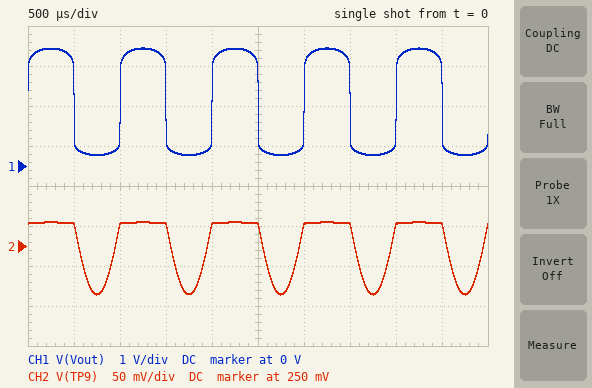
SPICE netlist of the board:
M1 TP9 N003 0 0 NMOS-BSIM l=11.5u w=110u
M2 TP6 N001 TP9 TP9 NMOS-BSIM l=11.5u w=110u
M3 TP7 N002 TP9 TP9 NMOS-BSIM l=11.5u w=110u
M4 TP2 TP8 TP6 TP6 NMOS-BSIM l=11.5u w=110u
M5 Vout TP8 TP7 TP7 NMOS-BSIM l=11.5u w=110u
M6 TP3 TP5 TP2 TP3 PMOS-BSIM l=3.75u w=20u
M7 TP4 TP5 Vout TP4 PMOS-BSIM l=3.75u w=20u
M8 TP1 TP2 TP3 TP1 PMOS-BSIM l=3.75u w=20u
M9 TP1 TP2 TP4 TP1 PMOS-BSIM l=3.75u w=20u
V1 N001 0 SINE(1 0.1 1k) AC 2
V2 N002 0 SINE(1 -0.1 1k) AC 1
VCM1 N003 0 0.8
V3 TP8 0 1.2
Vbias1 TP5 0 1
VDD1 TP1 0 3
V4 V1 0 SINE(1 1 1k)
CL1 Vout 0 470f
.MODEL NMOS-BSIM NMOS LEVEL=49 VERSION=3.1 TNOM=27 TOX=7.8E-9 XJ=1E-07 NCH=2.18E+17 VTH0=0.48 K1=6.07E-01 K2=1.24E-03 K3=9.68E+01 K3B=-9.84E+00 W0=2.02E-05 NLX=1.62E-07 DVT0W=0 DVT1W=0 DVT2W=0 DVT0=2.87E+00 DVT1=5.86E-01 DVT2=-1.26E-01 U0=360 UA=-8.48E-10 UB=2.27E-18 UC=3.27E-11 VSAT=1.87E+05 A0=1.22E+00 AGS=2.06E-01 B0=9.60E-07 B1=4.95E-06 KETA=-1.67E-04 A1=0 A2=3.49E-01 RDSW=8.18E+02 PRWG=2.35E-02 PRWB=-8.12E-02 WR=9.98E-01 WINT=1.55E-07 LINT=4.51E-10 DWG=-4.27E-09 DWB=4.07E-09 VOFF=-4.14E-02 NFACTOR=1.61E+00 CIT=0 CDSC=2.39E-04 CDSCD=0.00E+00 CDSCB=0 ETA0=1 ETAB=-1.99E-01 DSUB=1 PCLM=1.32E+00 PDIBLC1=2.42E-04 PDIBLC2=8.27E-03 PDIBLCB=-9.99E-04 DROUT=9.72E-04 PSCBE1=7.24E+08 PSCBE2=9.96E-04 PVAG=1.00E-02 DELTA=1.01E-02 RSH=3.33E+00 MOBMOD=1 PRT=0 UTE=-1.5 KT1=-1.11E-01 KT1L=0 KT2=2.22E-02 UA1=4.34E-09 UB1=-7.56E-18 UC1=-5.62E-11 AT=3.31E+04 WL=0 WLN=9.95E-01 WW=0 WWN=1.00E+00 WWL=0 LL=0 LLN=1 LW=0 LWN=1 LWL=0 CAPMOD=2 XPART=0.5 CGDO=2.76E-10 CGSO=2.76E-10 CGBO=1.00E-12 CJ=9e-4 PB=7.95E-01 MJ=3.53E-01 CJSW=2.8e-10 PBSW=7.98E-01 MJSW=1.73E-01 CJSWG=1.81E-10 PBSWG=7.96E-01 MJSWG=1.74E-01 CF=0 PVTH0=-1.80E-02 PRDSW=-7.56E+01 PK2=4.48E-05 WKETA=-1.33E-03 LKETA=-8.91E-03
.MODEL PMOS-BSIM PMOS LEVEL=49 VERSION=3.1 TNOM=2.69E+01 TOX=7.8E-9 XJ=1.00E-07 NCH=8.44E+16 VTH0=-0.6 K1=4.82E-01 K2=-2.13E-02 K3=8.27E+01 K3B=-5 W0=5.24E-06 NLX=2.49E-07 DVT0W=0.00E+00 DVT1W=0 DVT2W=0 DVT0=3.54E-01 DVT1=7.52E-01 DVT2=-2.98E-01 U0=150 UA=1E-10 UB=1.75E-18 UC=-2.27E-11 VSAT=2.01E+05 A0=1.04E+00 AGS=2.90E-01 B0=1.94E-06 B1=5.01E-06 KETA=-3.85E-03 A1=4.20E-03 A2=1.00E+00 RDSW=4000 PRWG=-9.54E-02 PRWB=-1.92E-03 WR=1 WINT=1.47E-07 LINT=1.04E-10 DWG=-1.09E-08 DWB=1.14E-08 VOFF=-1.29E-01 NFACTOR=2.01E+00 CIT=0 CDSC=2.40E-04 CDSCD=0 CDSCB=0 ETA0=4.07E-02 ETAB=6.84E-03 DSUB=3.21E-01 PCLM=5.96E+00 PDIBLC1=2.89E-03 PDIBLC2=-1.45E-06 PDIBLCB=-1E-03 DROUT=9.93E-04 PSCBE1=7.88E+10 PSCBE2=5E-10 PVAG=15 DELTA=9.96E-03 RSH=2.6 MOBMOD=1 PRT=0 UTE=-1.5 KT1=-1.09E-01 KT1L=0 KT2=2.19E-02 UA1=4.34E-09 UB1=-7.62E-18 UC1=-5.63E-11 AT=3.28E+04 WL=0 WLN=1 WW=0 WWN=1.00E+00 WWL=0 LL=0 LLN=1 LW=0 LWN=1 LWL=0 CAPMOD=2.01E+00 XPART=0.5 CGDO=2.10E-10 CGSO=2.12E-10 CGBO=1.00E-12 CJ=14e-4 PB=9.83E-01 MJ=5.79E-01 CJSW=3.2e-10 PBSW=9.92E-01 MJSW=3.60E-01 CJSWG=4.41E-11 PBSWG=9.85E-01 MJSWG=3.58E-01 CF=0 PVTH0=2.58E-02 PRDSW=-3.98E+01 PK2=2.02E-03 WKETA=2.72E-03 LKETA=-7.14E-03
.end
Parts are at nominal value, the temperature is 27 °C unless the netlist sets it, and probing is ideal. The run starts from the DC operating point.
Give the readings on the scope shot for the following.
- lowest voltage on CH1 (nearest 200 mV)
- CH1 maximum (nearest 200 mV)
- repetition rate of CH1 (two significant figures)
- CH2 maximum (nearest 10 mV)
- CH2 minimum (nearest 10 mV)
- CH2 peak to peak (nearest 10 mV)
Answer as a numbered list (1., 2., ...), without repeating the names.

1. 200 mV
2. 3.0 V
3. 1.0 kHz
4. 280 mV
5. 190 mV
6. 90 mV
